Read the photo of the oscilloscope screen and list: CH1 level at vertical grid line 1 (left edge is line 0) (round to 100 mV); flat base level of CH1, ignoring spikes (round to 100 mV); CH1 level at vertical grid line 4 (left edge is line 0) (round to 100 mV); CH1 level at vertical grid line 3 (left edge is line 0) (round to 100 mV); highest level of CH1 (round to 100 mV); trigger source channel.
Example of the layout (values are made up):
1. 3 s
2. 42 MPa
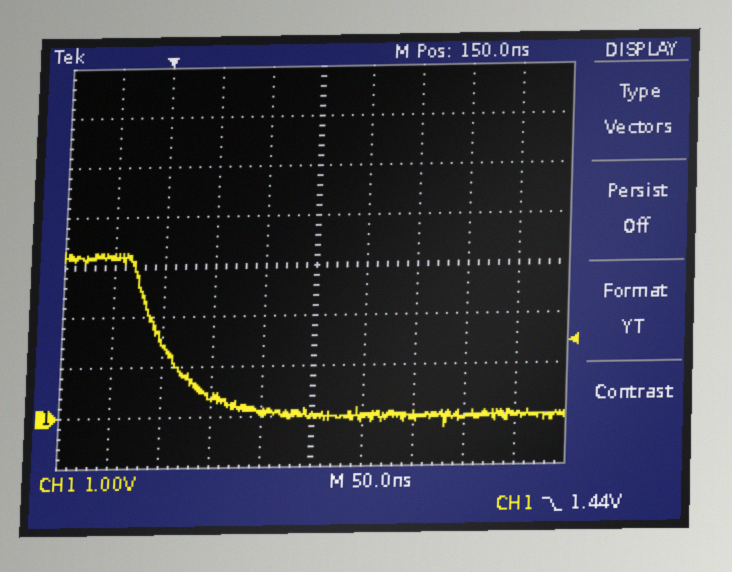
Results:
1. 3.2 V
2. 0.0 V
3. 100 mV
4. 400 mV
5. 3.3 V
6. CH1
